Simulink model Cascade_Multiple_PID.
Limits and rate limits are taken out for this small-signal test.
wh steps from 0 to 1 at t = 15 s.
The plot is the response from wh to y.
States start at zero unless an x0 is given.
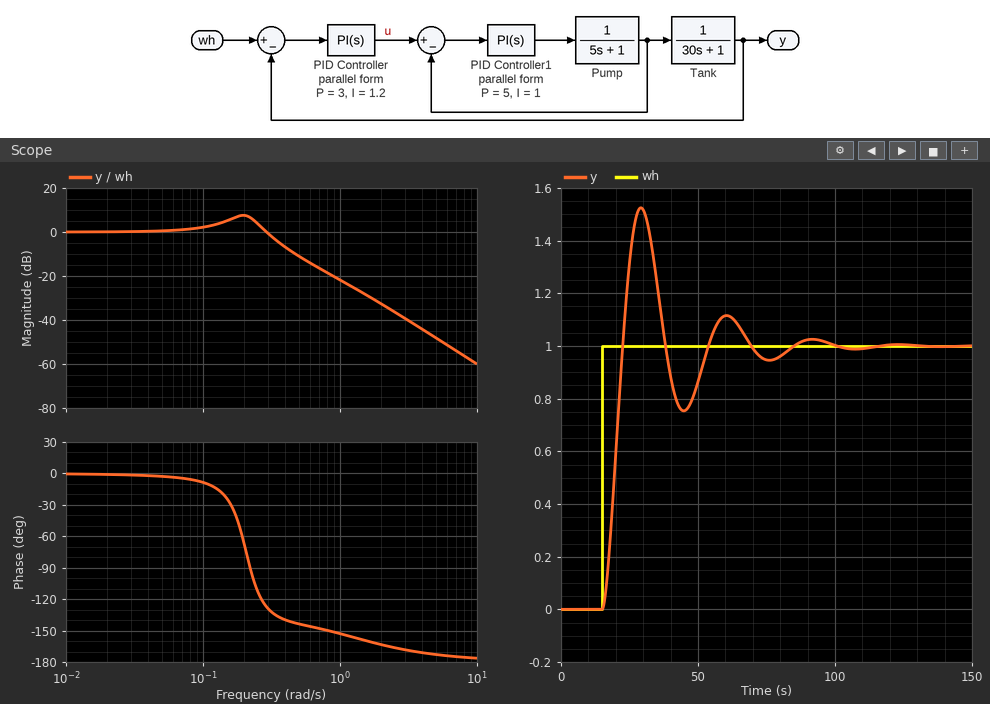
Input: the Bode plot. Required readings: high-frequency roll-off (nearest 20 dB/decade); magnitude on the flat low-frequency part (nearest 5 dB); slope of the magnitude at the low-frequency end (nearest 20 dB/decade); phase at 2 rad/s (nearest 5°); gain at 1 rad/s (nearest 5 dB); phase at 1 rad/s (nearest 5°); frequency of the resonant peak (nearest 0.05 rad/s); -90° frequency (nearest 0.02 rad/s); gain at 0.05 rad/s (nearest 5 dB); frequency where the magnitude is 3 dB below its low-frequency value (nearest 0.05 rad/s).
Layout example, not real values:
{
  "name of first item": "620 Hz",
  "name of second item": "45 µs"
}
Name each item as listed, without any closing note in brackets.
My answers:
{
  "high-frequency roll-off": "-40 dB/decade",
  "magnitude on the flat low-frequency part": "0 dB",
  "slope of the magnitude at the low-frequency end": "0 dB/decade",
  "phase at 2 rad/s": "-165°",
  "gain at 1 rad/s": "-20 dB",
  "phase at 1 rad/s": "-155°",
  "frequency of the resonant peak": "0.20 rad/s",
  "-90° frequency": "0.22 rad/s",
  "gain at 0.05 rad/s": "0 dB",
  "frequency where the magnitude is 3 dB below its low-frequency value": "0.35 rad/s"
}
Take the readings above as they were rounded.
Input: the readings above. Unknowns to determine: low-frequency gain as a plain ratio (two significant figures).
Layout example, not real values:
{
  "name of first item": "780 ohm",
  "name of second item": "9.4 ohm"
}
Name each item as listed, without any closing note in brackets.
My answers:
{
  "low-frequency gain as a plain ratio": "1.0"
}
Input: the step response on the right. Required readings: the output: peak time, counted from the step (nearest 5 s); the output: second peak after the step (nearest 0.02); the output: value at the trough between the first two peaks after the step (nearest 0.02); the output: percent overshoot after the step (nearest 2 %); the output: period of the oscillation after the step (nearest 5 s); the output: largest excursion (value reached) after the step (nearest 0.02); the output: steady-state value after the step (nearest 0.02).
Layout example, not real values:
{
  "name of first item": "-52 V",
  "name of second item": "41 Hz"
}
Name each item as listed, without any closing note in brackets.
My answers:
{
  "the output: peak time, counted from the step": "15 s",
  "the output: second peak after the step": "1.12",
  "the output: value at the trough between the first two peaks after the step": "0.76",
  "the output: percent overshoot after the step": "52 %",
  "the output: period of the oscillation after the step": "30 s",
  "the output: largest excursion (value reached) after the step": "1.52",
  "the output: steady-state value after the step": "1.00"
}
